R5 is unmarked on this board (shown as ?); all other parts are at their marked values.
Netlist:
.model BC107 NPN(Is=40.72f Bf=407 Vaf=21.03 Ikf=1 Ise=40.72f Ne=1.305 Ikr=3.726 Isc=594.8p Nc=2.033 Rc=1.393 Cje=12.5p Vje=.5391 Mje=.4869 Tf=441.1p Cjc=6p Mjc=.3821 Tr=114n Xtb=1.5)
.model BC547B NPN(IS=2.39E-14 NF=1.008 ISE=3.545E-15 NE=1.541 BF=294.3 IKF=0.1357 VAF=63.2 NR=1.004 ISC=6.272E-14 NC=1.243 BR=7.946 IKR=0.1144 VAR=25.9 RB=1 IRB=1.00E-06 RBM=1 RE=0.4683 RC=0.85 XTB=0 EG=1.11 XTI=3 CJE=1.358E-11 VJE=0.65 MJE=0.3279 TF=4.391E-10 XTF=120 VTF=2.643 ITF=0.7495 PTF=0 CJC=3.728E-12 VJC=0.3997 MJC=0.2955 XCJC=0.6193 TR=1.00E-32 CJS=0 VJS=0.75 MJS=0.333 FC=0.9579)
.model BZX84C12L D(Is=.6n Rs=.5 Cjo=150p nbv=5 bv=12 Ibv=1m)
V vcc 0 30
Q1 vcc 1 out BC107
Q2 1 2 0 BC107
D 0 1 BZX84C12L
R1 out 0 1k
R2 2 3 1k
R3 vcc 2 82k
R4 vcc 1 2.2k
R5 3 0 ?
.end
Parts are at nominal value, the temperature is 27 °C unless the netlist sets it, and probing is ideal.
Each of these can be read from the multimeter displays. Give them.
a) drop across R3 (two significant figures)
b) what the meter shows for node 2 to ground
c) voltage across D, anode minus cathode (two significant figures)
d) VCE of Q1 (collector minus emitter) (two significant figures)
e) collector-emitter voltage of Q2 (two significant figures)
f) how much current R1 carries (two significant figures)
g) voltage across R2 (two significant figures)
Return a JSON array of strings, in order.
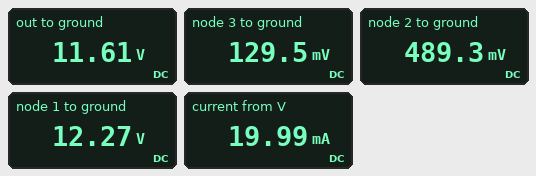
["30 V", "489.3 mV", "-12 V", "18 V", "12 V", "12 mA", "360 mV"]
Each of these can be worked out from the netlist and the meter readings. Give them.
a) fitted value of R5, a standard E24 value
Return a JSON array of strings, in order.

["360 Ω"]
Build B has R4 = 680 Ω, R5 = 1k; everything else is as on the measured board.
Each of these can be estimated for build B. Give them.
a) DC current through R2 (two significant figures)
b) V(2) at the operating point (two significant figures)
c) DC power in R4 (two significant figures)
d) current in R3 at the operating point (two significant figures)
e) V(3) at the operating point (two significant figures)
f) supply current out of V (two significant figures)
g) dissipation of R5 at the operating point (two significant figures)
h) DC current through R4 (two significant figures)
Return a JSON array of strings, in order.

["330 µA", "660 mV", "460 mW", "360 µA", "330 mV", "38 mA", "110 µW", "26 mA"]
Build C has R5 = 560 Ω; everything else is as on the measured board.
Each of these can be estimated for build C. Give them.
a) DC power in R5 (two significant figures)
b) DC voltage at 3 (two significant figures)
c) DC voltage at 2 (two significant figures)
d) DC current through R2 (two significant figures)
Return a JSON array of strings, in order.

["72 µW", "200 mV", "560 mV", "360 µA"]
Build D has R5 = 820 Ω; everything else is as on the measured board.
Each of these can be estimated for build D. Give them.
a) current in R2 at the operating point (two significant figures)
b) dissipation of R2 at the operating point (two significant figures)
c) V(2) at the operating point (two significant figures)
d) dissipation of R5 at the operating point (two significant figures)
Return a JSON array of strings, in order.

["350 µA", "120 µW", "630 mV", "99 µW"]
